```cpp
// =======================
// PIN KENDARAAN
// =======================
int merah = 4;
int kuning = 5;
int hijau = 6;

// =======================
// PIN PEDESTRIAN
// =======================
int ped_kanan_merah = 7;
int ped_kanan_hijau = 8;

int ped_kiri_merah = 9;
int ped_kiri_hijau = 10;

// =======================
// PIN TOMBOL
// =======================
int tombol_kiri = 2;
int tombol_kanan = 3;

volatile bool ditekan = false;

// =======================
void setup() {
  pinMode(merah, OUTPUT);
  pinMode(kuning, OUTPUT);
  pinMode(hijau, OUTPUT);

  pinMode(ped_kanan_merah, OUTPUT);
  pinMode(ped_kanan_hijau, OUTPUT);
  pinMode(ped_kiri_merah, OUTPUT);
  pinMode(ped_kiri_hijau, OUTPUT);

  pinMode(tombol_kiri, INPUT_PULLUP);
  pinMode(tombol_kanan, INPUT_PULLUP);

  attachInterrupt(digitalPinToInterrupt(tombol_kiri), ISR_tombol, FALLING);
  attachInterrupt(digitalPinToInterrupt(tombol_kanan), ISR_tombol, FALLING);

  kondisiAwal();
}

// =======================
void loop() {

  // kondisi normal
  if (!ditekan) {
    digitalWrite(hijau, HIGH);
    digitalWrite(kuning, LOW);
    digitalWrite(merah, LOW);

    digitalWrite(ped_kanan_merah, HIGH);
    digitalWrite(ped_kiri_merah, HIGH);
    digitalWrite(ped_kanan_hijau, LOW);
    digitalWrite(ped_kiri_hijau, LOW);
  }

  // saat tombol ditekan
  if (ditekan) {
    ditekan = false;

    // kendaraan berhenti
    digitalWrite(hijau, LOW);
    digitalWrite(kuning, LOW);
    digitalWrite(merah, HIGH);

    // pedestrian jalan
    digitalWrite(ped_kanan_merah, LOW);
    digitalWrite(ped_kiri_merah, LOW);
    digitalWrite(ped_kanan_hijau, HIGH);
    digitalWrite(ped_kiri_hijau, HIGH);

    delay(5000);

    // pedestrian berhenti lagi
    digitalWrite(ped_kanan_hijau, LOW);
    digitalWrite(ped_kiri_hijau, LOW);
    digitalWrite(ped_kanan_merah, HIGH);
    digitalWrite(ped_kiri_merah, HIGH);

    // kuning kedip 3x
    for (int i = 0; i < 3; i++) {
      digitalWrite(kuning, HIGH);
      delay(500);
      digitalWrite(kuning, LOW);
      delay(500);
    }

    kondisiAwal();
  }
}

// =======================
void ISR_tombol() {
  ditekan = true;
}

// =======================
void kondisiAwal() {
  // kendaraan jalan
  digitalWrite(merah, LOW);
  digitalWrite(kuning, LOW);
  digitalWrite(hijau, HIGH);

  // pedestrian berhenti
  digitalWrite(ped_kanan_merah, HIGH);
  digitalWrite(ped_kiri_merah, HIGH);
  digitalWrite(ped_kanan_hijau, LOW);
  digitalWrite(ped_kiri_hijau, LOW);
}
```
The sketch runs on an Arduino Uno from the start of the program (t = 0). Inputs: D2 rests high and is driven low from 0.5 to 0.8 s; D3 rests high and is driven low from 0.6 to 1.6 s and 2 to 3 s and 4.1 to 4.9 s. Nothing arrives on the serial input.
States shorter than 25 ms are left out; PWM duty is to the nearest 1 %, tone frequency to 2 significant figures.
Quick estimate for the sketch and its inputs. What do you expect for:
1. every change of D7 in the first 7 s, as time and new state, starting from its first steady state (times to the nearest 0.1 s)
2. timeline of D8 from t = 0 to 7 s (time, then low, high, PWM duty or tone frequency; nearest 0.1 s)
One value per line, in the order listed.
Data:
0 s high; 0.5 s low; 5.5 s high
0 s low; 0.5 s high; 5.5 s low
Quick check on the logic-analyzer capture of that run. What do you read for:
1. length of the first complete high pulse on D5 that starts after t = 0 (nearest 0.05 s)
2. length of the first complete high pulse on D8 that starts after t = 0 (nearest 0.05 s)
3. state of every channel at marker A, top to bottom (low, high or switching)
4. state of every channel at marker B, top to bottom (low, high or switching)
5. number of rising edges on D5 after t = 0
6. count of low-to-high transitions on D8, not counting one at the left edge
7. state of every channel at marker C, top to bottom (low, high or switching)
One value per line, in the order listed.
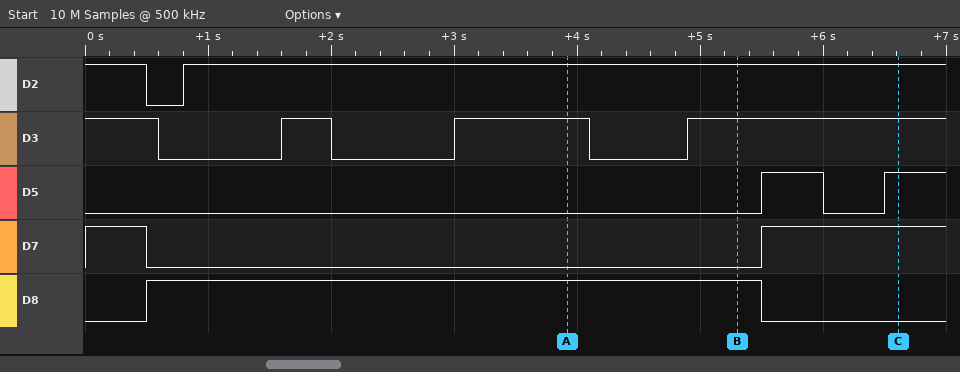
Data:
0.50 s
5.00 s
D2 high, D3 high, D5 low, D7 low, D8 high
D2 high, D3 high, D5 low, D7 low, D8 high
2
1
D2 high, D3 high, D5 high, D7 high, D8 low
